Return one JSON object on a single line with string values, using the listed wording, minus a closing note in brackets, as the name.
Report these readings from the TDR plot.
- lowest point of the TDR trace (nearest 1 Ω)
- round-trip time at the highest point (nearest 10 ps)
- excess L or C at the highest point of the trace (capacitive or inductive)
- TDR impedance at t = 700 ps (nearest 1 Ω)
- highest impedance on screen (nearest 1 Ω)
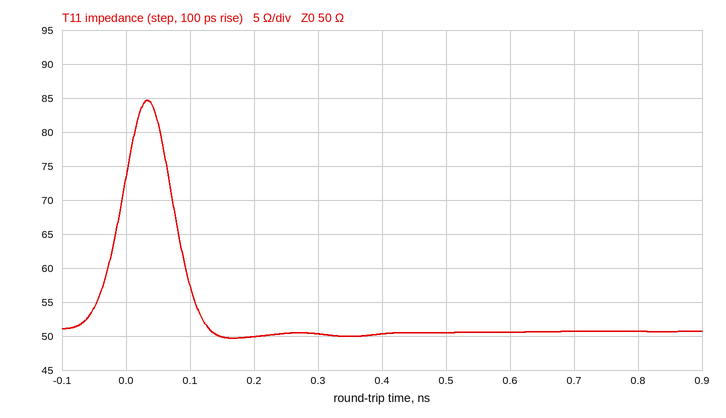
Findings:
{"lowest point of the TDR trace": "50 Ω", "round-trip time at the highest point": "30 ps", "excess L or C at the highest point of the trace": "inductive", "TDR impedance at t = 700 ps": "51 Ω", "highest impedance on screen": "85 Ω"}
